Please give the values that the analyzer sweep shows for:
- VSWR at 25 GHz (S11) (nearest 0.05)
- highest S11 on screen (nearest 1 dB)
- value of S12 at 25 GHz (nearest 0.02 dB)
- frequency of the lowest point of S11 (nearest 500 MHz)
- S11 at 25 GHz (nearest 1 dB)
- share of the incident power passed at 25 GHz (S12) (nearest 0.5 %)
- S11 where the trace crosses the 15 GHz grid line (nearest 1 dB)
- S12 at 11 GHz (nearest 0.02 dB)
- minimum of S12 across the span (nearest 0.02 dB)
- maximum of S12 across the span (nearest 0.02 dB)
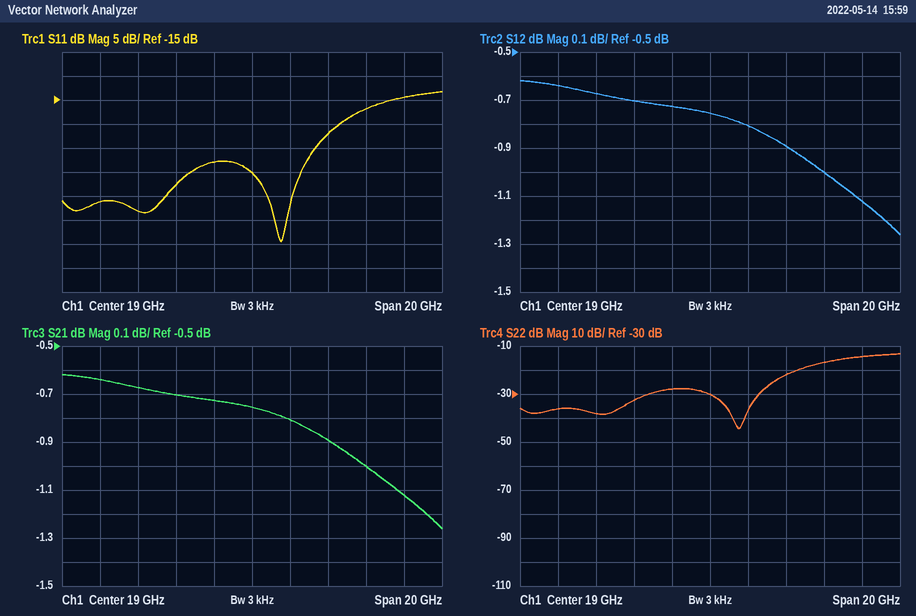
1.35
-13 dB
-1.00 dB
20.5 GHz
-17 dB
79.5 %
-33 dB
-0.64 dB
-1.26 dB
-0.62 dB
